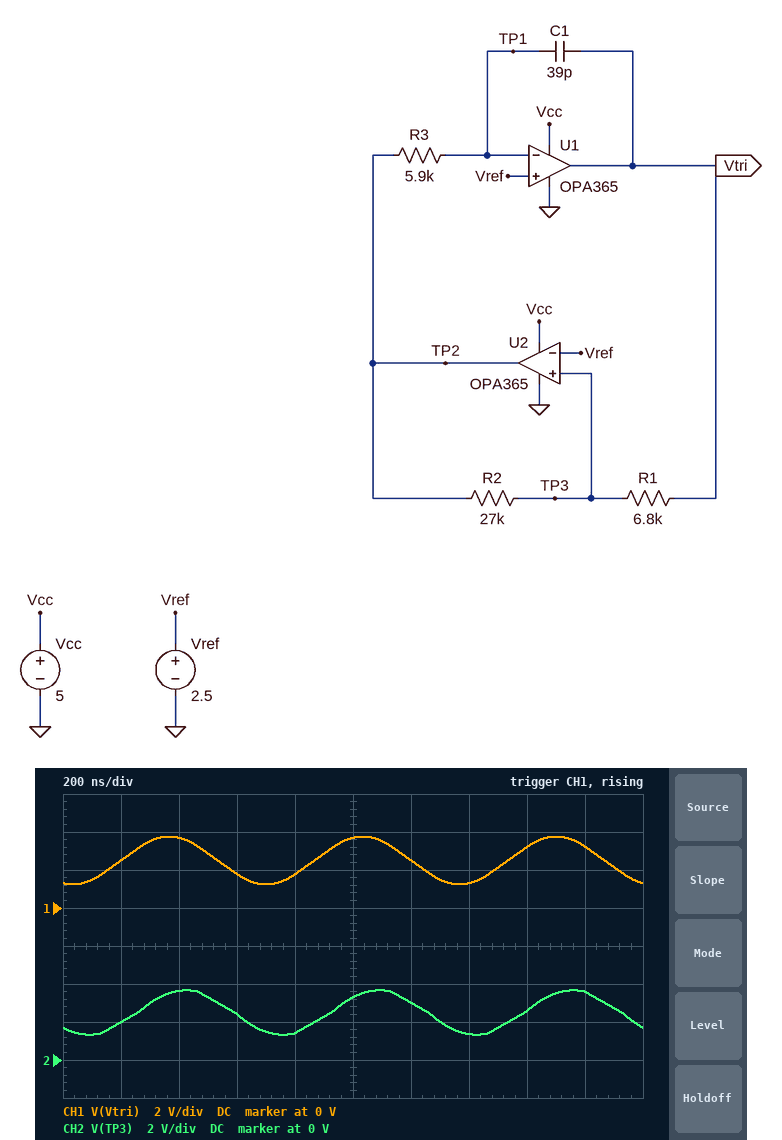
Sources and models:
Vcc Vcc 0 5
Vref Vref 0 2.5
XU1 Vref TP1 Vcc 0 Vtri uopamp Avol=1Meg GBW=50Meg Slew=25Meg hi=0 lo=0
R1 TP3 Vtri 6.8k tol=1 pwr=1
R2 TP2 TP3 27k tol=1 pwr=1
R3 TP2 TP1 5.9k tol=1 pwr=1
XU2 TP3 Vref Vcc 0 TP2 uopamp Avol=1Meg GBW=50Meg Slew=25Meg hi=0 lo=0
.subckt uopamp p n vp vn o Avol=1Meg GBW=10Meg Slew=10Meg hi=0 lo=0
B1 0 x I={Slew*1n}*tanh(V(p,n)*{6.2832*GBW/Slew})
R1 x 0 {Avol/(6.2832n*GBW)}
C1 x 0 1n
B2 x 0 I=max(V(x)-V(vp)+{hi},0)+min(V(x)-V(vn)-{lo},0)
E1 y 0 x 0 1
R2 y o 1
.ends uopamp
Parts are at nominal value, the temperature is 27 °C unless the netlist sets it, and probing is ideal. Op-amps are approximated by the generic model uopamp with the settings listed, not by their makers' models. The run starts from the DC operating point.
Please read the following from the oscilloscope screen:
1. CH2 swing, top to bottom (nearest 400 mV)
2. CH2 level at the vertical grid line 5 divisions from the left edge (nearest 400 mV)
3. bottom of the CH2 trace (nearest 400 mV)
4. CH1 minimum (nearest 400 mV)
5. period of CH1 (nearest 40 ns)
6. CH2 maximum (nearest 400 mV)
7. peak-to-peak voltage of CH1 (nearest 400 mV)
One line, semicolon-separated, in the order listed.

2.4 V; 3.2 V; 1.2 V; 1.2 V; 680 ns; 3.6 V; 2.4 V
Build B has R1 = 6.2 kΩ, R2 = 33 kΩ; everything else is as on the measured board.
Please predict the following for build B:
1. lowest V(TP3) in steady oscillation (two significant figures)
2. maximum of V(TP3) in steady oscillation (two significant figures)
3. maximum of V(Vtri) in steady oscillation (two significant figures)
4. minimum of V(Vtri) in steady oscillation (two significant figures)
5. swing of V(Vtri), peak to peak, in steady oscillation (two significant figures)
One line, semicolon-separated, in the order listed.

1.5 V; 3.5 V; 3.6 V; 1.4 V; 2.2 V
